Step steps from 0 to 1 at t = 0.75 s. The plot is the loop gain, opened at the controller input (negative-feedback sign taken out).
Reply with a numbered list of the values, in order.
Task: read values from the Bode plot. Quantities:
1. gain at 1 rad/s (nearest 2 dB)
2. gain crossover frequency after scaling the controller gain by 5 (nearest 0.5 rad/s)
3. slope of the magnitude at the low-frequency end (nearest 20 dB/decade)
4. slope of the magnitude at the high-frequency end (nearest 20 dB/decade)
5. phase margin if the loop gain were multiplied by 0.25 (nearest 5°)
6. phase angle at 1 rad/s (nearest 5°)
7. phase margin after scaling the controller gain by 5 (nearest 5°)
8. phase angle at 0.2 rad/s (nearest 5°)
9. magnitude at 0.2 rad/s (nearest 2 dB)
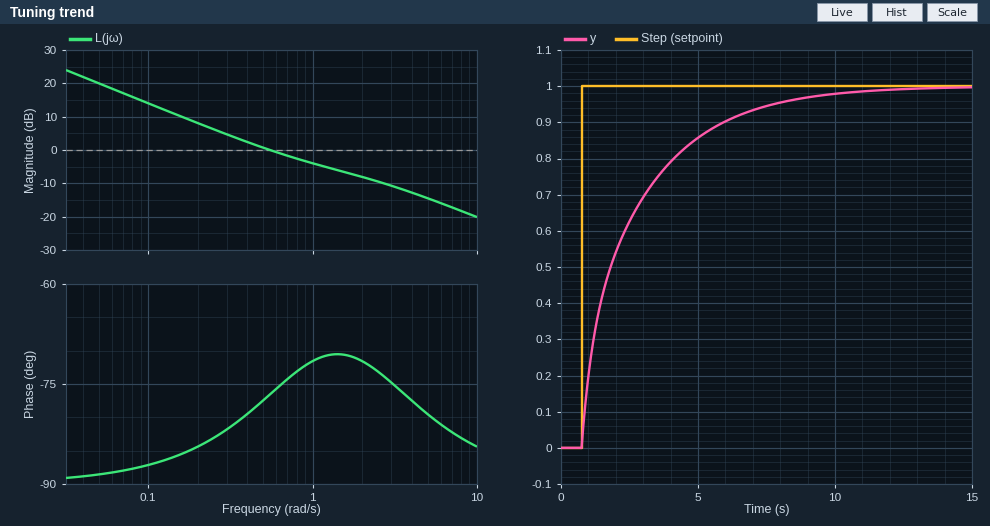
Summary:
1. -4 dB
2. 4.5 rad/s
3. -20 dB/decade
4. -20 dB/decade
5. 95°
6. -70°
7. 100°
8. -85°
9. 8 dB
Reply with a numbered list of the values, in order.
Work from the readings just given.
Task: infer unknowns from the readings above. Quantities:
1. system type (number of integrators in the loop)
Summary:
1. 1
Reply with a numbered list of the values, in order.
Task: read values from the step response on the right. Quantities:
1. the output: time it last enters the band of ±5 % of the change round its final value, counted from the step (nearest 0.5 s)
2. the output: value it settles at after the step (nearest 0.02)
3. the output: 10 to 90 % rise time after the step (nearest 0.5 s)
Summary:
1. 7.0 s
2. 1.00
3. 5.0 s
